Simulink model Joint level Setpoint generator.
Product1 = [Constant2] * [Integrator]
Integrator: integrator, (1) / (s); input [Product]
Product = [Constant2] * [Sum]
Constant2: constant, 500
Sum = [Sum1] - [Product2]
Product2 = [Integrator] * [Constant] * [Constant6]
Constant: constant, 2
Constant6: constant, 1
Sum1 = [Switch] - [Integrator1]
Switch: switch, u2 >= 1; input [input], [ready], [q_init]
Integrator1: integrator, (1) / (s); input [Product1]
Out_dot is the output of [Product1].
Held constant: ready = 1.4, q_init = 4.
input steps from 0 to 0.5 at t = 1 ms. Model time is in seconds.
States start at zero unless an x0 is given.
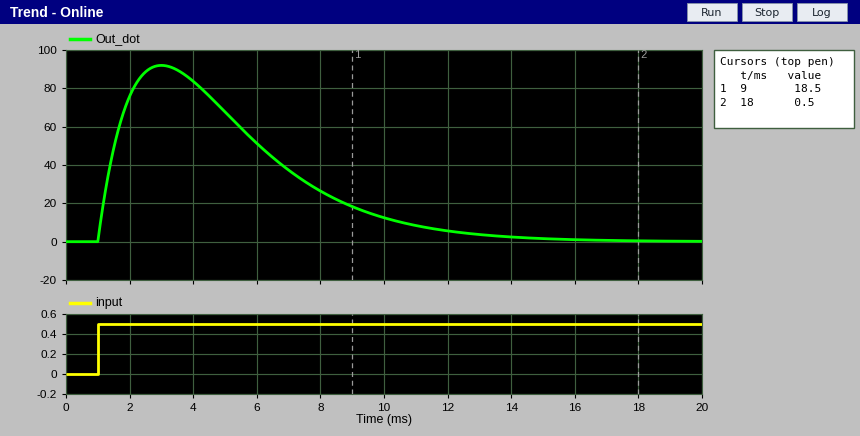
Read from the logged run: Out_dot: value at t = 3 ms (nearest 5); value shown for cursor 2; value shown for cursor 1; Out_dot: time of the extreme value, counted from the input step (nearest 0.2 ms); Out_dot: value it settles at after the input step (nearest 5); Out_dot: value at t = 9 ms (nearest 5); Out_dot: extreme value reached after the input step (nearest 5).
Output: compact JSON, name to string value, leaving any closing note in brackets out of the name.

{"Out_dot: value at t = 3 ms": "90", "value shown for cursor 2": "0.5", "value shown for cursor 1": "18.5", "Out_dot: time of the extreme value, counted from the input step": "2.0 ms", "Out_dot: value it settles at after the input step": "0", "Out_dot: value at t = 9 ms": "20", "Out_dot: extreme value reached after the input step": "90"}
